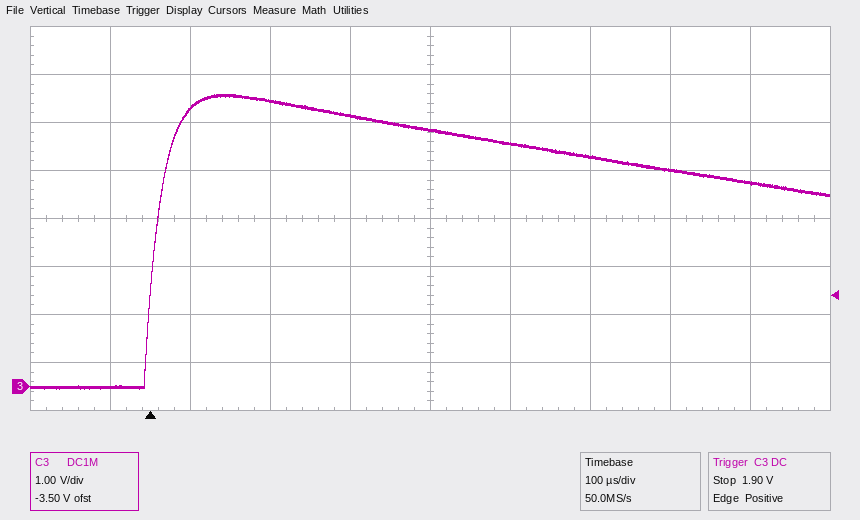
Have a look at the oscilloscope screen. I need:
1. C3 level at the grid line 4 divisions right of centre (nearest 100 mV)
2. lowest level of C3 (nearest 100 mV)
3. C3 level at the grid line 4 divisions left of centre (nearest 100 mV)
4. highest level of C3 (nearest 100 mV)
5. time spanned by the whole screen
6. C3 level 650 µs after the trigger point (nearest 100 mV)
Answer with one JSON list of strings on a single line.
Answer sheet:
["4.2 V", "-100 mV", "0.0 V", "6.1 V", "1 ms", "4.5 V"]
